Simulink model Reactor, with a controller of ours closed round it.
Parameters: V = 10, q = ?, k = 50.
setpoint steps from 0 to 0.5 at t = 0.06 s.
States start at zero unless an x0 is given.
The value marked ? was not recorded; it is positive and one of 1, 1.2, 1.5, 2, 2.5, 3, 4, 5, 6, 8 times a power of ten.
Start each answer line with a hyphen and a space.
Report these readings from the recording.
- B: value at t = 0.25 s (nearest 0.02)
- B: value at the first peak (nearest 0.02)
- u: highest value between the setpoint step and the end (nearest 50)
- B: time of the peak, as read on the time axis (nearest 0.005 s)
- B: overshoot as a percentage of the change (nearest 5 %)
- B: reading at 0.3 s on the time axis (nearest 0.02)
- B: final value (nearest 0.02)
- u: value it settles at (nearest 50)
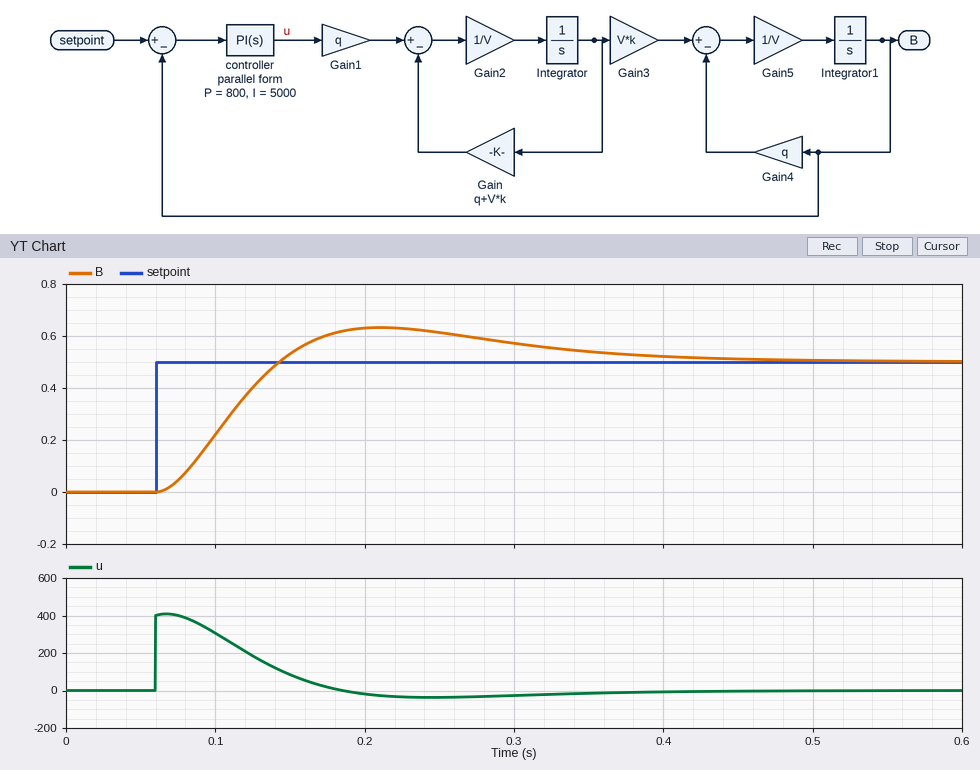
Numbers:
- 0.62
- 0.64
- 400
- 0.210 s
- 25 %
- 0.58
- 0.50
- 0
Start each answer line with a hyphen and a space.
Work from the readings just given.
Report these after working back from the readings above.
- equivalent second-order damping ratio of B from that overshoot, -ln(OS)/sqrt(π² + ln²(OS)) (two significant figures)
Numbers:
- 0.40
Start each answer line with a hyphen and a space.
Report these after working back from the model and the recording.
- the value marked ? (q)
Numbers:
- 0.25
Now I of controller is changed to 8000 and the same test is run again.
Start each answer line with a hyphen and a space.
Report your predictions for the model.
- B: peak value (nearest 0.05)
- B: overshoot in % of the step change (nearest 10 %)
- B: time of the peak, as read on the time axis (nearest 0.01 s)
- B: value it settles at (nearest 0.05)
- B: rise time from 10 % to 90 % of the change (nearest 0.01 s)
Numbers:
- 0.70
- 40 %
- 0.20 s
- 0.50
- 0.05 s
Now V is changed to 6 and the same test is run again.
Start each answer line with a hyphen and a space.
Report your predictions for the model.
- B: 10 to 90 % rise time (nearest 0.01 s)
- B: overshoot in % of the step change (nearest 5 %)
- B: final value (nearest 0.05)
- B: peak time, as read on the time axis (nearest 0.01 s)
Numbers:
- 0.04 s
- 30 %
- 0.50
- 0.16 s
